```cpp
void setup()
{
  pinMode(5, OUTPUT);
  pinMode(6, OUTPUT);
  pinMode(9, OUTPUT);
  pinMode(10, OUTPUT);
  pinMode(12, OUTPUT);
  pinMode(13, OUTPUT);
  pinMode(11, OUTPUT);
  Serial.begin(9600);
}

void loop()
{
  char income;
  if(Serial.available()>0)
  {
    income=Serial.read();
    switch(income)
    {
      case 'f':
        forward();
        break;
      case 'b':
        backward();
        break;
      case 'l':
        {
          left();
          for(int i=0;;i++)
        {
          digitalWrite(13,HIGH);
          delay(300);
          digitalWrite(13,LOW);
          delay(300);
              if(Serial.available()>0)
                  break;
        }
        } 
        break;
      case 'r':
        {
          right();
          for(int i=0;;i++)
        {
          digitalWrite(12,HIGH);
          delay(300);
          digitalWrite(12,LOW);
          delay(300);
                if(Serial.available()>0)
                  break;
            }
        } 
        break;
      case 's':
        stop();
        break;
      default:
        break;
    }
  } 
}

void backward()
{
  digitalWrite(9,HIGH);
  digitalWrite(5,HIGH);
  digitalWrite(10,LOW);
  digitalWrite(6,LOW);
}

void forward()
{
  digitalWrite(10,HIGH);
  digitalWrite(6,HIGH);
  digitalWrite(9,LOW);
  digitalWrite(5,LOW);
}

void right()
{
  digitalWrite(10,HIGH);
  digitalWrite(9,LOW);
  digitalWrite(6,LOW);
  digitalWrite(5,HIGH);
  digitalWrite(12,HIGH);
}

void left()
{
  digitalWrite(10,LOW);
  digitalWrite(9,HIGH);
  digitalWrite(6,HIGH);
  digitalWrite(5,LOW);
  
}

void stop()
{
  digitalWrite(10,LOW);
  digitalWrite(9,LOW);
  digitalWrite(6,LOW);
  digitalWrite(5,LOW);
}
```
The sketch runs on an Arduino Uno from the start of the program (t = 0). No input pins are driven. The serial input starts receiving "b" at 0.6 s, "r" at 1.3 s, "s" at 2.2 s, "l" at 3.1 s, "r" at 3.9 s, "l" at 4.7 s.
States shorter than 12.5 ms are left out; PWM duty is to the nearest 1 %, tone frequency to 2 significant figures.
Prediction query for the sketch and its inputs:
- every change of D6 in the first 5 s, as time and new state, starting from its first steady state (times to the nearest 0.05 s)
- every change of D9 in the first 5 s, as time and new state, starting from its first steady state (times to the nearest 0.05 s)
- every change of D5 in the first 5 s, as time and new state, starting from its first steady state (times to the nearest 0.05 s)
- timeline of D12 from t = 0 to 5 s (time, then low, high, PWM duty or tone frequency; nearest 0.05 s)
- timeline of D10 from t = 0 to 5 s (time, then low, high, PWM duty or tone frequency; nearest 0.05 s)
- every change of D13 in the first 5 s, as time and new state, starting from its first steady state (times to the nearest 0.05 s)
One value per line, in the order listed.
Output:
0 s low; 3.1 s high; 4.3 s low; 4.9 s high
0 s low; 0.6 s high; 1.3 s low; 3.1 s high; 4.3 s low; 4.9 s high
0 s low; 0.6 s high; 2.5 s low; 4.3 s high; 4.9 s low
0 s low; 1.3 s high; 1.6 s low; 1.9 s high; 2.2 s low; 4.3 s high; 4.6 s low
0 s low; 1.3 s high; 2.5 s low; 4.3 s high; 4.9 s low
0 s low; 3.1 s high; 3.4 s low; 3.7 s high; 4 s low; 4.9 s high
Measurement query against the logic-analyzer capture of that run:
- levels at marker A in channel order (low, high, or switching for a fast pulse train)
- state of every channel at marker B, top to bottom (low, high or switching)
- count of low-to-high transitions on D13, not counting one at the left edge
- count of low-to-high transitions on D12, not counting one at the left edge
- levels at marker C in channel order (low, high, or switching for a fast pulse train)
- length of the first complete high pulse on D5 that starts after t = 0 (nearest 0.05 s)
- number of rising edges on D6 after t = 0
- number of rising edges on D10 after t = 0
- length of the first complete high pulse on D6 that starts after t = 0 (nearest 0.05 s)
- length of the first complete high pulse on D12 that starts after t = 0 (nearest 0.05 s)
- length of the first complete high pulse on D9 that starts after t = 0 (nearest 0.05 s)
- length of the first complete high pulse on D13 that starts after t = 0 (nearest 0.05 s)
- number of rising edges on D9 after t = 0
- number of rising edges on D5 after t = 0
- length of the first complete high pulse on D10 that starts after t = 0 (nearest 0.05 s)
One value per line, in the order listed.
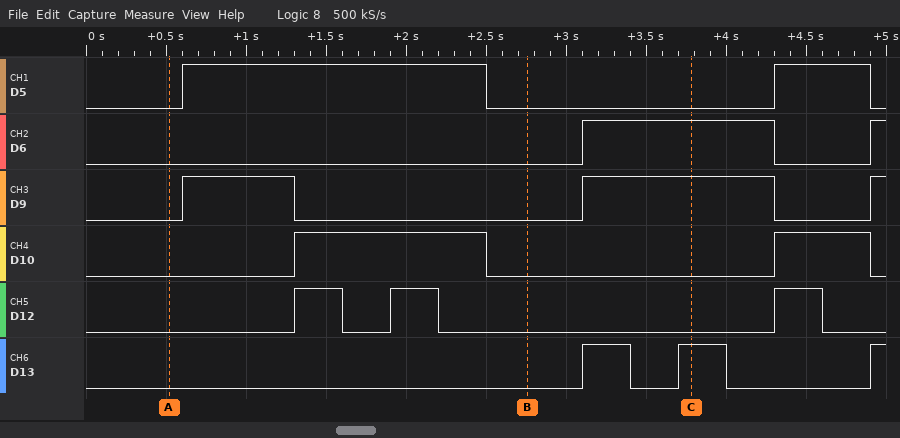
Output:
D5 low, D6 low, D9 low, D10 low, D12 low, D13 low
D5 low, D6 low, D9 low, D10 low, D12 low, D13 low
3
3
D5 low, D6 high, D9 high, D10 low, D12 low, D13 high
1.90 s
2
2
1.20 s
0.30 s
0.70 s
0.30 s
3
2
1.20 s
